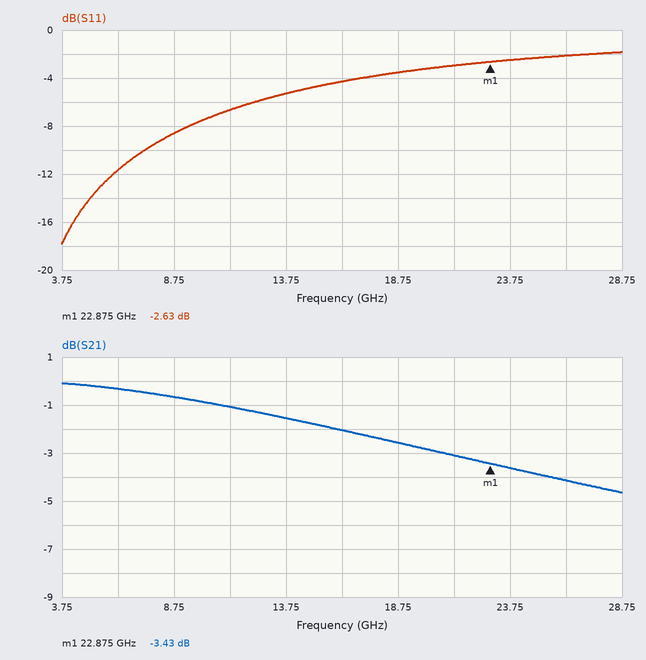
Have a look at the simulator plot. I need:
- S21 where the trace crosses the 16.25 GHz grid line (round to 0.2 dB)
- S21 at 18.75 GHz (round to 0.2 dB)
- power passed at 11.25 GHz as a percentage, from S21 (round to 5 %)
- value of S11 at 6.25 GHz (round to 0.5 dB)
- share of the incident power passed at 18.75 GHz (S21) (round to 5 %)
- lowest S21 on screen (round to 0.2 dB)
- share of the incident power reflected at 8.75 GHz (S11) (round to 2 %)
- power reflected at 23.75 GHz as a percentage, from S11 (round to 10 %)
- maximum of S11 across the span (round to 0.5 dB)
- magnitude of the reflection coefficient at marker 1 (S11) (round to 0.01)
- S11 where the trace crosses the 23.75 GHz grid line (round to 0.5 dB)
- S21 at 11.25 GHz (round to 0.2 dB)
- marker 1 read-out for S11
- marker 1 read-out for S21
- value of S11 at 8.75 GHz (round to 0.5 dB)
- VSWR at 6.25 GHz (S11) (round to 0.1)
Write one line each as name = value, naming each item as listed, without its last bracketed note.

S21 where the trace crosses the 16.25 GHz grid line = -2.0 dB
S21 at 18.75 GHz = -2.6 dB
power passed at 11.25 GHz as a percentage, from S21 = 80 %
value of S11 at 6.25 GHz = -11.5 dB
share of the incident power passed at 18.75 GHz (S21) = 55 %
lowest S21 on screen = -4.6 dB
share of the incident power reflected at 8.75 GHz (S11) = 14 %
power reflected at 23.75 GHz as a percentage, from S11 = 60 %
maximum of S11 across the span = -2.0 dB
magnitude of the reflection coefficient at marker 1 (S11) = 0.74
S11 where the trace crosses the 23.75 GHz grid line = -2.5 dB
S21 at 11.25 GHz = -1.0 dB
marker 1 read-out for S11 = -2.63 dB
marker 1 read-out for S21 = -3.43 dB
value of S11 at 8.75 GHz = -8.5 dB
VSWR at 6.25 GHz (S11) = 1.7
